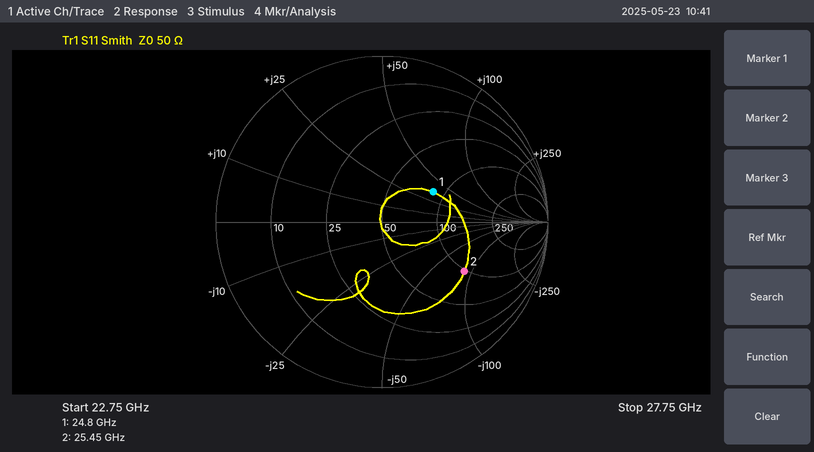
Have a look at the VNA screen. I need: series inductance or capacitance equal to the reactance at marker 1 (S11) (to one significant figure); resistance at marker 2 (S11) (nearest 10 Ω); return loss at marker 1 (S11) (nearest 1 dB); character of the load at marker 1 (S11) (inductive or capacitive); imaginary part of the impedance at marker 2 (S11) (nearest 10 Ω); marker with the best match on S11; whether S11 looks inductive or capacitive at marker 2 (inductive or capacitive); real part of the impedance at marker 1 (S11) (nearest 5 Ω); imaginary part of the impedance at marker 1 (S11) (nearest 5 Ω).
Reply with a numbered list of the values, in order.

1. 200 pH
2. 100 Ω
3. 9 dB
4. inductive
5. -90 Ω
6. marker 1
7. capacitive
8. 85 Ω
9. +35 Ω
